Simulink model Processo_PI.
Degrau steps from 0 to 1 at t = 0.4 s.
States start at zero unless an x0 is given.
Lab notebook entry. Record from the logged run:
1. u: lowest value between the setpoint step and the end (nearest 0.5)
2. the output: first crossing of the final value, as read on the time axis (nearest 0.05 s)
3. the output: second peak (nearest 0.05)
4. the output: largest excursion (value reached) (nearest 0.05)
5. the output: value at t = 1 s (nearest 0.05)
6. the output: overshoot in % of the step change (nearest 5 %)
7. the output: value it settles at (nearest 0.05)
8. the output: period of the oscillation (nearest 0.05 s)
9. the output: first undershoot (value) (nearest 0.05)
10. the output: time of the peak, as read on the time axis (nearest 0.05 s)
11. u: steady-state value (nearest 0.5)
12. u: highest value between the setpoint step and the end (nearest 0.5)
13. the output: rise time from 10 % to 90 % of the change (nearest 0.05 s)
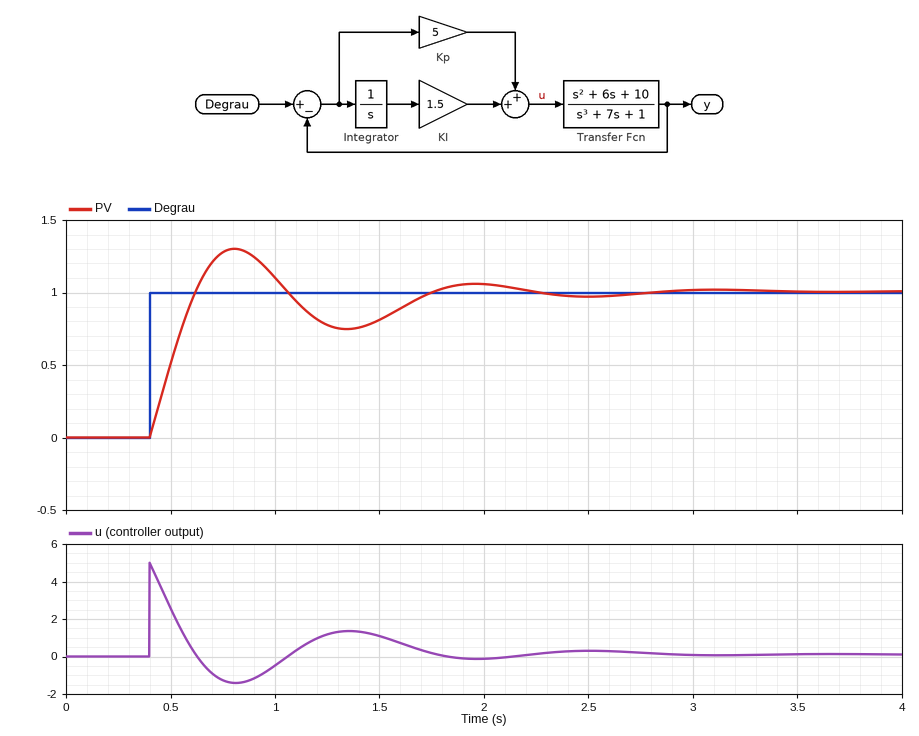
-1.5
0.60 s
1.05
1.30
1.10
30 %
1.00
1.15 s
0.75
0.80 s
0.0
5.0
0.15 s
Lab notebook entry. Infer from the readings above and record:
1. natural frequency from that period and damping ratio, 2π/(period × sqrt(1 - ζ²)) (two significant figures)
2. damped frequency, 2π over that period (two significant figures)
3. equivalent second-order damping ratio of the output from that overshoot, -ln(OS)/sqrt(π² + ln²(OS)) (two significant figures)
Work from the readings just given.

5.9 rad/s
5.5 rad/s
0.36
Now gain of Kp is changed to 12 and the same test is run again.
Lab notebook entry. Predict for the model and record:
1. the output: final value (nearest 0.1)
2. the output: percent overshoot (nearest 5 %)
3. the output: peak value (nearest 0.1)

1.0
20 %
1.2
